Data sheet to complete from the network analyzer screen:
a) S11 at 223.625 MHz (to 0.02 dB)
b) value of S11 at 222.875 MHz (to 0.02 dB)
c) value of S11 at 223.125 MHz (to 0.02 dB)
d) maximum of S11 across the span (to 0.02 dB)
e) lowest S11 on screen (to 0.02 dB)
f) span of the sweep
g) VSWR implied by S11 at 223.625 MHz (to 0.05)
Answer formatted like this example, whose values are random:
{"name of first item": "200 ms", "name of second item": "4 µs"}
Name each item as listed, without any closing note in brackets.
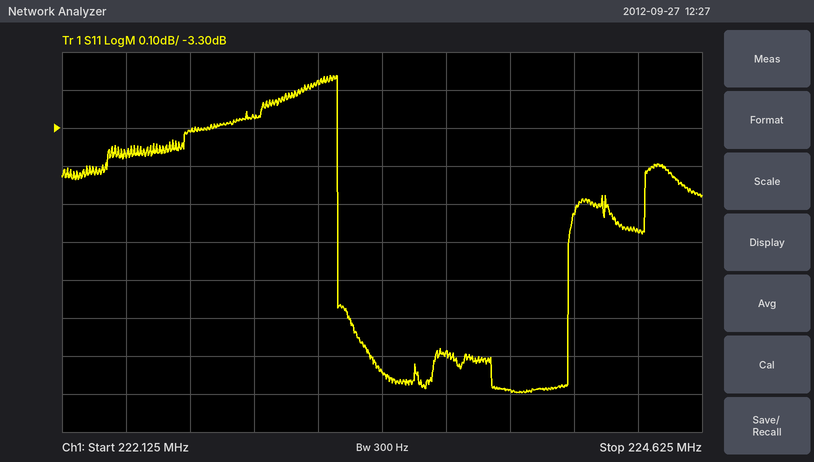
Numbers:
{"S11 at 223.625 MHz": "-3.88 dB", "value of S11 at 222.875 MHz": "-3.28 dB", "value of S11 at 223.125 MHz": "-3.18 dB", "maximum of S11 across the span": "-3.16 dB", "lowest S11 on screen": "-4.00 dB", "span of the sweep": "2.5 MHz", "VSWR implied by S11 at 223.625 MHz": "4.55"}
